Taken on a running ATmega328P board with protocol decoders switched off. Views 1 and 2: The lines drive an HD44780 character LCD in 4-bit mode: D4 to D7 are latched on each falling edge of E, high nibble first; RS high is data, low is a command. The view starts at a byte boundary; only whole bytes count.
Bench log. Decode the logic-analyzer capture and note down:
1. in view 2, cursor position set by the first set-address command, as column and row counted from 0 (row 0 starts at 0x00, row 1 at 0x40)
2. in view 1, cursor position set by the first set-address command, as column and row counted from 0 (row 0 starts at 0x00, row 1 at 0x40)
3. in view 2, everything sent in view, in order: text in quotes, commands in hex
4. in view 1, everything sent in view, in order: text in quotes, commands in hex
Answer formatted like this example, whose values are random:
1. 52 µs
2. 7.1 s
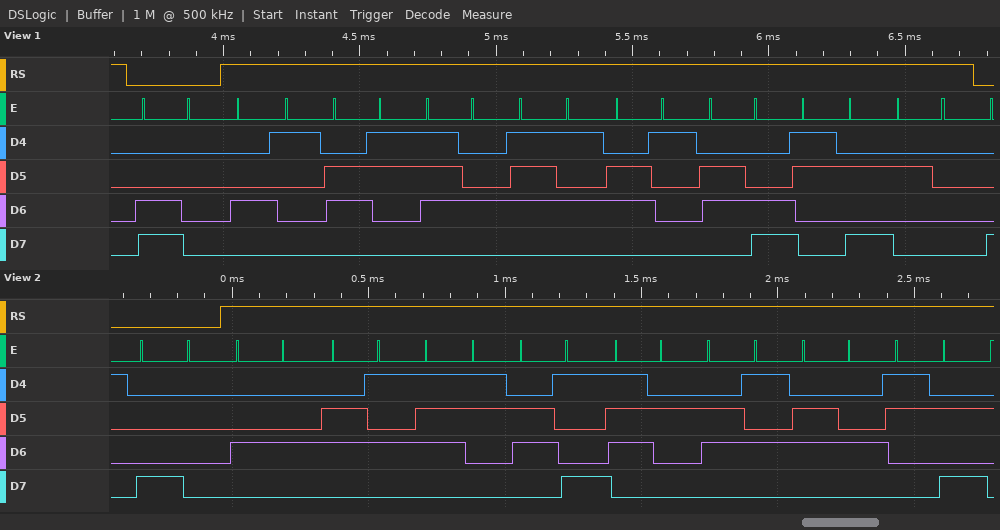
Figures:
1. column 0, row 0
2. column 0, row 1
3. 0x80 "Desired:"
4. 0xC0 "Actual: "
